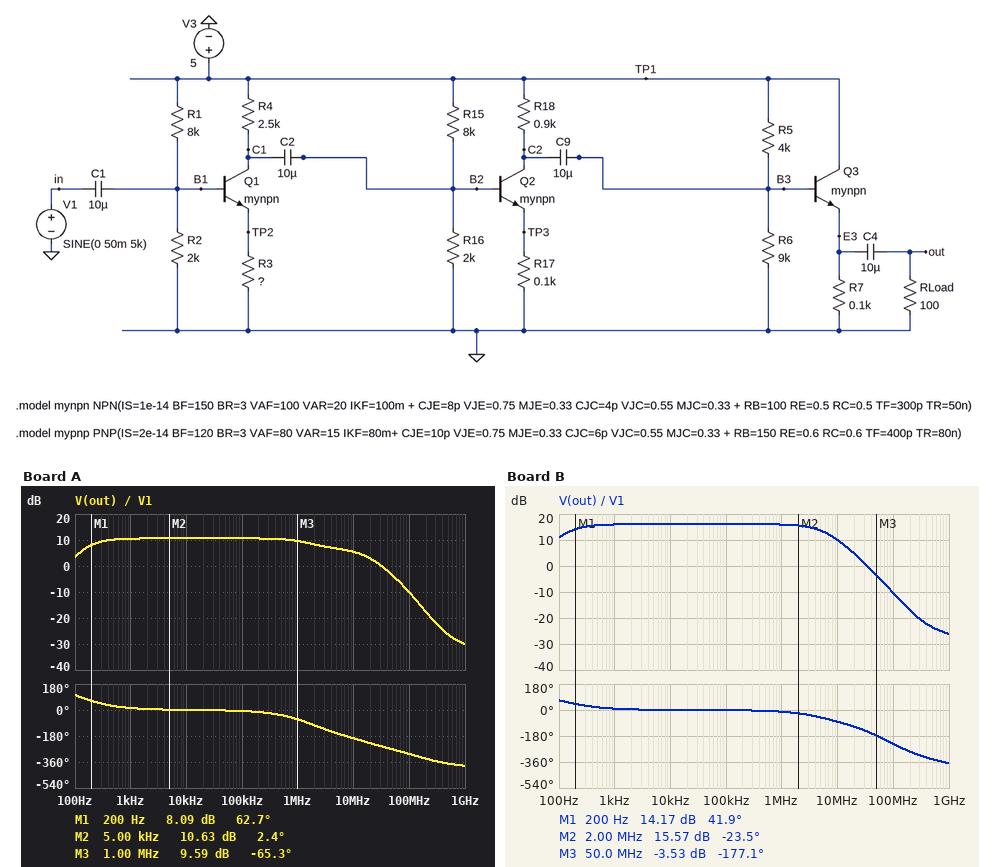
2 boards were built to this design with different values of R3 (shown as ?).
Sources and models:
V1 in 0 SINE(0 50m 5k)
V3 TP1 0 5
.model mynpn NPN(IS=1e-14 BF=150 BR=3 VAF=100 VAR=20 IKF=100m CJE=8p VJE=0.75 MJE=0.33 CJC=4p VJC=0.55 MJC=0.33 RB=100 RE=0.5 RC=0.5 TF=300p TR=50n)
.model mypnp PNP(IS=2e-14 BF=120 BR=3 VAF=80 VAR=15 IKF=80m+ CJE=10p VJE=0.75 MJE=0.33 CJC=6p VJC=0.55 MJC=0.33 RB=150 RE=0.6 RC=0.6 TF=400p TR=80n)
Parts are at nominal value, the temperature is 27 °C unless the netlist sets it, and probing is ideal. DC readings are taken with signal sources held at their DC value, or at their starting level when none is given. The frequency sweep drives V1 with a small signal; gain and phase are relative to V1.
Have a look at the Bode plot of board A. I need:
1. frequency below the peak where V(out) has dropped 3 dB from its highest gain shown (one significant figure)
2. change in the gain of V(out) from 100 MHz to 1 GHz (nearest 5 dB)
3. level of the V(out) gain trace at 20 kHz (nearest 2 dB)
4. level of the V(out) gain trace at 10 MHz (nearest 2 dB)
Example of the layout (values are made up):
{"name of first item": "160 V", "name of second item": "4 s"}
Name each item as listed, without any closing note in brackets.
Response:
{"frequency below the peak where V(out) has dropped 3 dB from its highest gain shown": "200 Hz", "change in the gain of V(out) from 100 MHz to 1 GHz": "-20 dB", "level of the V(out) gain trace at 20 kHz": "10 dB", "level of the V(out) gain trace at 10 MHz": "6 dB"}
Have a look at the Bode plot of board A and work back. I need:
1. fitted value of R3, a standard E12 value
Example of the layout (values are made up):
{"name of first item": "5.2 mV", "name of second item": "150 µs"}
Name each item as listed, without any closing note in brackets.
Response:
{"fitted value of R3, a standard E12 value": "68 Ω"}
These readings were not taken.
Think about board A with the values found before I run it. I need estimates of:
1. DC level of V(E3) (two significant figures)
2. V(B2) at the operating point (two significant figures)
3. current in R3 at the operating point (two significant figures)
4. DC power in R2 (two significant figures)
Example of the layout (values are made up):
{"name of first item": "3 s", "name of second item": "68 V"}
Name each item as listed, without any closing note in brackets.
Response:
{"DC level of V(E3)": "2.2 V", "V(B2) at the operating point": "970 mV", "current in R3 at the operating point": "2.0 mA", "DC power in R2": "340 µW"}
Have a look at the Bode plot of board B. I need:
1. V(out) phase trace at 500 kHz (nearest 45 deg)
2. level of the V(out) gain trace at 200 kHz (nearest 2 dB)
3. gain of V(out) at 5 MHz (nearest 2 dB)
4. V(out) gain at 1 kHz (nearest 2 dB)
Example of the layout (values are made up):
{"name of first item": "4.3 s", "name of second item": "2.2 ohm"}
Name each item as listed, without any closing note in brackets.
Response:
{"V(out) phase trace at 500 kHz": "0 deg", "level of the V(out) gain trace at 200 kHz": "16 dB", "gain of V(out) at 5 MHz": "14 dB", "V(out) gain at 1 kHz": "16 dB"}
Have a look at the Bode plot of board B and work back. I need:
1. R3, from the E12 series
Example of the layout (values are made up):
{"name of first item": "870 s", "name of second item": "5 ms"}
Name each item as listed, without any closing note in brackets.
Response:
{"R3, from the E12 series": "680 Ω"}
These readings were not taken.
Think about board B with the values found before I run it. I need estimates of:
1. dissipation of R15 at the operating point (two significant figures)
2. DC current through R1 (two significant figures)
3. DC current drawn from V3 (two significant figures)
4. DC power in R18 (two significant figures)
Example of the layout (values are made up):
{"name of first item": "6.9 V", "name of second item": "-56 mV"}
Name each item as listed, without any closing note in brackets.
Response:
{"dissipation of R15 at the operating point": "2.0 mW", "DC current through R1": "500 µA", "DC current drawn from V3": "27 mA", "DC power in R18": "7.1 mW"}
